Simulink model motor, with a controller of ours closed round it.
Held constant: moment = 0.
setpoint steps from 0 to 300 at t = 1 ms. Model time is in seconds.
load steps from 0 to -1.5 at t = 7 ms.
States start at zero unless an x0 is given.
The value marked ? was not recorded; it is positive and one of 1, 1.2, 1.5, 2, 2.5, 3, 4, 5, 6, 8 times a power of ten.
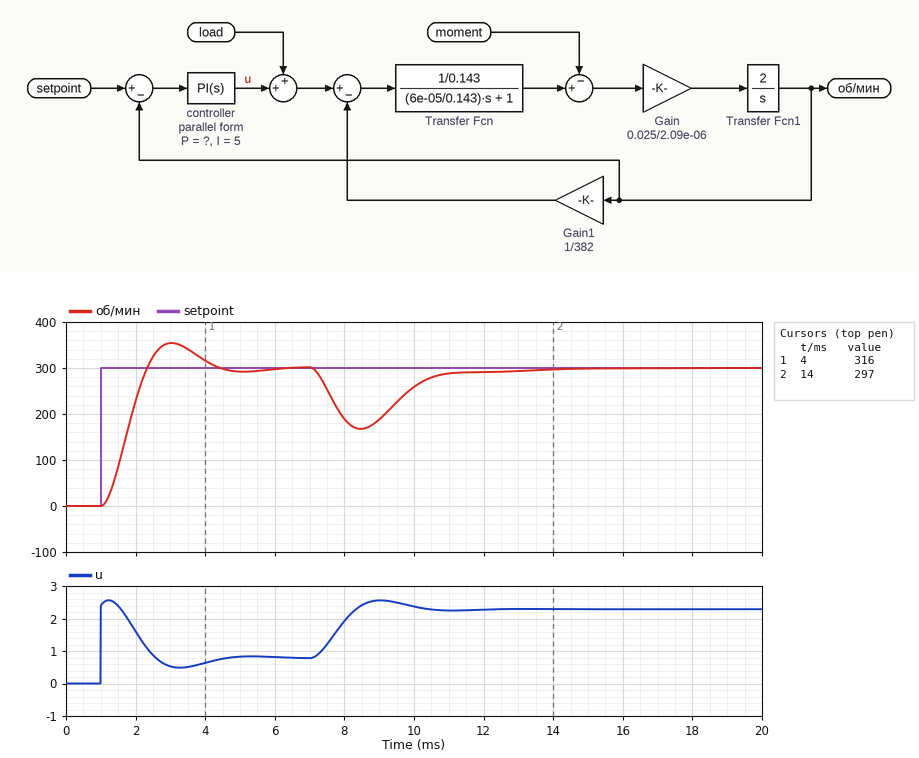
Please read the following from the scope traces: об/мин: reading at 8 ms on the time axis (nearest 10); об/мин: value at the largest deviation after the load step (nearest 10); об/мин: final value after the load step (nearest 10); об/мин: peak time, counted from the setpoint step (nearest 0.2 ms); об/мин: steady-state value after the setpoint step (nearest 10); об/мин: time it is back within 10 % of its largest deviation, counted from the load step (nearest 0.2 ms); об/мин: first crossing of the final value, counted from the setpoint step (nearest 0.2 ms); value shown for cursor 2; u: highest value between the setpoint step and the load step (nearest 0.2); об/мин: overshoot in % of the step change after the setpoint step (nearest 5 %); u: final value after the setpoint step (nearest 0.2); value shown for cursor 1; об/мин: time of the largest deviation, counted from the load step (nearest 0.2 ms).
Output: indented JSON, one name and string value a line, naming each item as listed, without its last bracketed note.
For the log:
{
  "об/мин: reading at 8 ms on the time axis": "190",
  "об/мин: value at the largest deviation after the load step": "170",
  "об/мин: final value after the load step": "300",
  "об/мин: peak time, counted from the setpoint step": "2.0 ms",
  "об/мин: steady-state value after the setpoint step": "300",
  "об/мин: time it is back within 10 % of its largest deviation, counted from the load step": "3.8 ms",
  "об/мин: first crossing of the final value, counted from the setpoint step": "1.4 ms",
  "value shown for cursor 2": "297",
  "u: highest value between the setpoint step and the load step": "2.6",
  "об/мин: overshoot in % of the step change after the setpoint step": "20 %",
  "u: final value after the setpoint step": "0.8",
  "value shown for cursor 1": "316",
  "об/мин: time of the largest deviation, counted from the load step": "1.4 ms"
}
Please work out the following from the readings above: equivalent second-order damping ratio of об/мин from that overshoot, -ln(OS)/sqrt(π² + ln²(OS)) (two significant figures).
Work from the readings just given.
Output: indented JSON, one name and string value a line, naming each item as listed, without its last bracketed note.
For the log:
{
  "equivalent second-order damping ratio of об/мин from that overshoot, -ln(OS)/sqrt(π² + ln²(OS))": "0.46"
}
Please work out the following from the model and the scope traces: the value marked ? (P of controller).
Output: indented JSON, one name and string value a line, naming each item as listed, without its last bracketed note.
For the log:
{
  "the value marked ?": "0.008"
}
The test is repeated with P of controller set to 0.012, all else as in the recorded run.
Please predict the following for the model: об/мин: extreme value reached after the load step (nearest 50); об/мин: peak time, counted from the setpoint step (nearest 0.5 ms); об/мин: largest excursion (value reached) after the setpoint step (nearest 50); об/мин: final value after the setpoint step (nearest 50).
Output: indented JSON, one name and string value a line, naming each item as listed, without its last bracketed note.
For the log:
{
  "об/мин: extreme value reached after the load step": "200",
  "об/мин: peak time, counted from the setpoint step": "1.5 ms",
  "об/мин: largest excursion (value reached) after the setpoint step": "350",
  "об/мин: final value after the setpoint step": "300"
}
